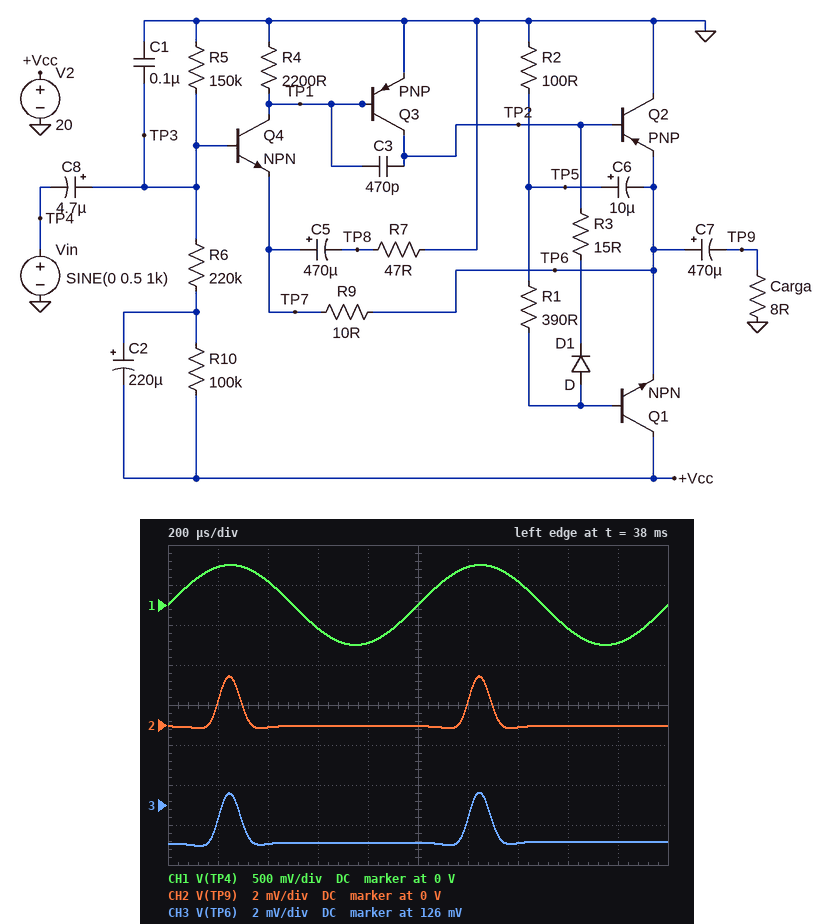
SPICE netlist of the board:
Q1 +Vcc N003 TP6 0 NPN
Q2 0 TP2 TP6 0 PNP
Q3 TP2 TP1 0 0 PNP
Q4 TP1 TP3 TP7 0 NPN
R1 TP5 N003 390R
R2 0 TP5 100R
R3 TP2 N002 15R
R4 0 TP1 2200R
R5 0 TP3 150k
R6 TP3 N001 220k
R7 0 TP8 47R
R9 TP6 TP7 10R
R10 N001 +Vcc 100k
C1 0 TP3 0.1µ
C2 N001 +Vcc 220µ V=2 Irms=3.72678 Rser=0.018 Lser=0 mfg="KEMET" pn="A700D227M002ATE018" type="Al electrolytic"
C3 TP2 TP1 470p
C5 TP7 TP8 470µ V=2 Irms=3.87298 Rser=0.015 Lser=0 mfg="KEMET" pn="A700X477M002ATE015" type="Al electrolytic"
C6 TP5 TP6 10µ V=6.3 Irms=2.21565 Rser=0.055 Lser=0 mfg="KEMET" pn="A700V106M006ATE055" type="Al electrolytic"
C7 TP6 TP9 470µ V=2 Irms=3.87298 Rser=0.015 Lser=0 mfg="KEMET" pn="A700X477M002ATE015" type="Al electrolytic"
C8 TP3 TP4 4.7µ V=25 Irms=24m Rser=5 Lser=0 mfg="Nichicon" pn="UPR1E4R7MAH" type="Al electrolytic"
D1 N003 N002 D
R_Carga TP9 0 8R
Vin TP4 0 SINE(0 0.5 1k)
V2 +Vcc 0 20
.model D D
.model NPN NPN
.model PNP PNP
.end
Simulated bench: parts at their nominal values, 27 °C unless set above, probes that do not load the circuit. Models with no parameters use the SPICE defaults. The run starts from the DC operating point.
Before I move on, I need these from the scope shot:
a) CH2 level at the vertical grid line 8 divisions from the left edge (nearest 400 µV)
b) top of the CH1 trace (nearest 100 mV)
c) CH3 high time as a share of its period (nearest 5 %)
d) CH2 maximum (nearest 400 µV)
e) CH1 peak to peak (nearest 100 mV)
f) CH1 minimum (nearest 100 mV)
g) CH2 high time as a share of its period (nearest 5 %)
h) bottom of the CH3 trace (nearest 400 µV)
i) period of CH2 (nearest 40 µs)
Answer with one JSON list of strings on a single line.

["0 V", "500 mV", "10 %", "2.4 mV", "1.0 V", "-500 mV", "10 %", "124.0 mV", "1.00 ms"]
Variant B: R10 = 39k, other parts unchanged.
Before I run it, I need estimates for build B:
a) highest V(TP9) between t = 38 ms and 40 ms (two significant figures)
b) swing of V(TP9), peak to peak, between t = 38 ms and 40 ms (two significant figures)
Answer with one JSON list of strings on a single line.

["2.9 mV", "3.1 mV"]
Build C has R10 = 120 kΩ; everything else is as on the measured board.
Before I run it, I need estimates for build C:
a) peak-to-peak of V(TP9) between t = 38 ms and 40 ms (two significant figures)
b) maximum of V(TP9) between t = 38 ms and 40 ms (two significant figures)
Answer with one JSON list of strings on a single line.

["2.5 mV", "2.3 mV"]
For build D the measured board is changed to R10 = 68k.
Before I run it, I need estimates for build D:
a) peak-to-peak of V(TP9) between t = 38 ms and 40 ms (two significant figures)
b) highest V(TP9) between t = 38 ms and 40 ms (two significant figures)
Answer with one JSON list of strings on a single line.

["2.9 mV", "2.7 mV"]
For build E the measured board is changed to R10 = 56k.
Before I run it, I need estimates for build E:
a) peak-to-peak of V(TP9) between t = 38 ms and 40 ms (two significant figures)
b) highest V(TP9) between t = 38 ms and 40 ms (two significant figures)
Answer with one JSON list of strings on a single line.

["3.0 mV", "2.8 mV"]
